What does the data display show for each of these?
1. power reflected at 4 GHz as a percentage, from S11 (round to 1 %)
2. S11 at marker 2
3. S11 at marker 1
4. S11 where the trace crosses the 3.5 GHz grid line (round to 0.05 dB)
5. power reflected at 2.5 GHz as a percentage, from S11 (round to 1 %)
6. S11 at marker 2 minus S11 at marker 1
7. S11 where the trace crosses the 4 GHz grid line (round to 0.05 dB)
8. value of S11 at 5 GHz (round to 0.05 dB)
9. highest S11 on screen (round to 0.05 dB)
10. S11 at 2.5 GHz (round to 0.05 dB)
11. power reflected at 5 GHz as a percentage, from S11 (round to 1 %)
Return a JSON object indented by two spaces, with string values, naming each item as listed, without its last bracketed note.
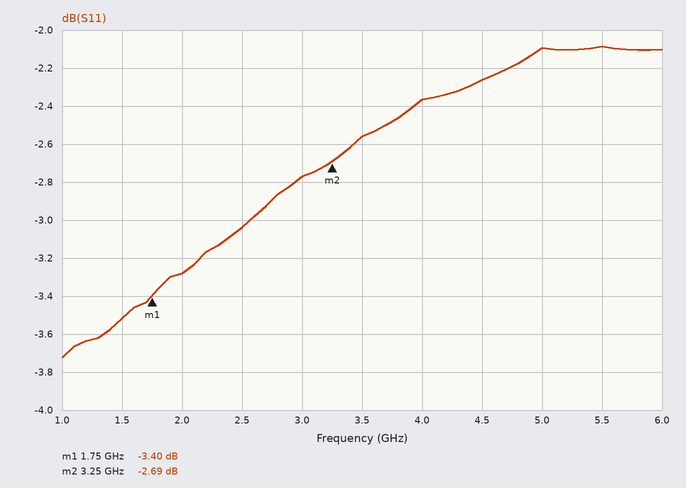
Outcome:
{
  "power reflected at 4 GHz as a percentage, from S11": "58 %",
  "S11 at marker 2": "-2.69 dB",
  "S11 at marker 1": "-3.40 dB",
  "S11 where the trace crosses the 3.5 GHz grid line": "-2.55 dB",
  "power reflected at 2.5 GHz as a percentage, from S11": "50 %",
  "S11 at marker 2 minus S11 at marker 1": "0.71 dB",
  "S11 where the trace crosses the 4 GHz grid line": "-2.35 dB",
  "value of S11 at 5 GHz": "-2.10 dB",
  "highest S11 on screen": "-2.10 dB",
  "S11 at 2.5 GHz": "-3.05 dB",
  "power reflected at 5 GHz as a percentage, from S11": "62 %"
}
